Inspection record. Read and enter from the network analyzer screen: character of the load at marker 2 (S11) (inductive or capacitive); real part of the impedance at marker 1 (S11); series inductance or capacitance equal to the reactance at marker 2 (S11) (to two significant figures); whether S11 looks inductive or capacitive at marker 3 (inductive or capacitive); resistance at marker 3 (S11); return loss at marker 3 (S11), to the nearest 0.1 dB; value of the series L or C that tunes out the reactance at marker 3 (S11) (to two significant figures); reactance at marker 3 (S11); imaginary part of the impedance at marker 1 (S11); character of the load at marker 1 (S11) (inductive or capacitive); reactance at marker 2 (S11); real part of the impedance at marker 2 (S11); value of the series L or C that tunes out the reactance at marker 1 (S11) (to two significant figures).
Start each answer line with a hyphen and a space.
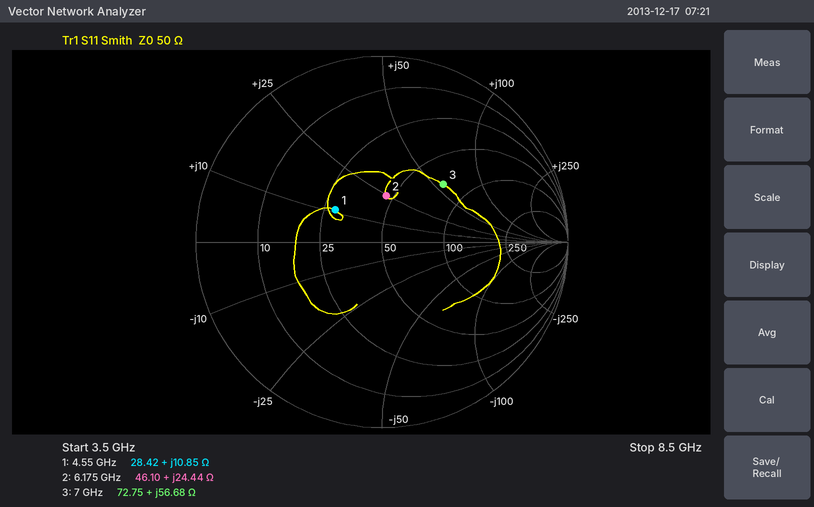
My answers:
- inductive
- 28.42 Ω
- 630 pH
- inductive
- 72.75 Ω
- 6.9 dB
- 400 fF
- +56.68 Ω
- +10.85 Ω
- inductive
- +24.44 Ω
- 46.10 Ω
- 3.2 pF
